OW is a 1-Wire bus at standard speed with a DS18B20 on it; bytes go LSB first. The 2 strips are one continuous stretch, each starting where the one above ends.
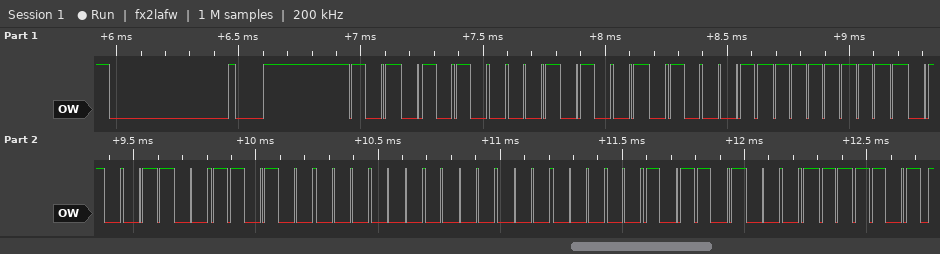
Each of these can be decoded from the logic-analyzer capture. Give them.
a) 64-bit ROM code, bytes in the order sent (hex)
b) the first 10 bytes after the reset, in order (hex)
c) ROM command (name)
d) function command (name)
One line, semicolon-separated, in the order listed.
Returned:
28 C5 FF 32 0B 00 00 2D; 55 28 C5 FF 32 0B 00 00 2D BE; Match ROM; Read Scratchpad
